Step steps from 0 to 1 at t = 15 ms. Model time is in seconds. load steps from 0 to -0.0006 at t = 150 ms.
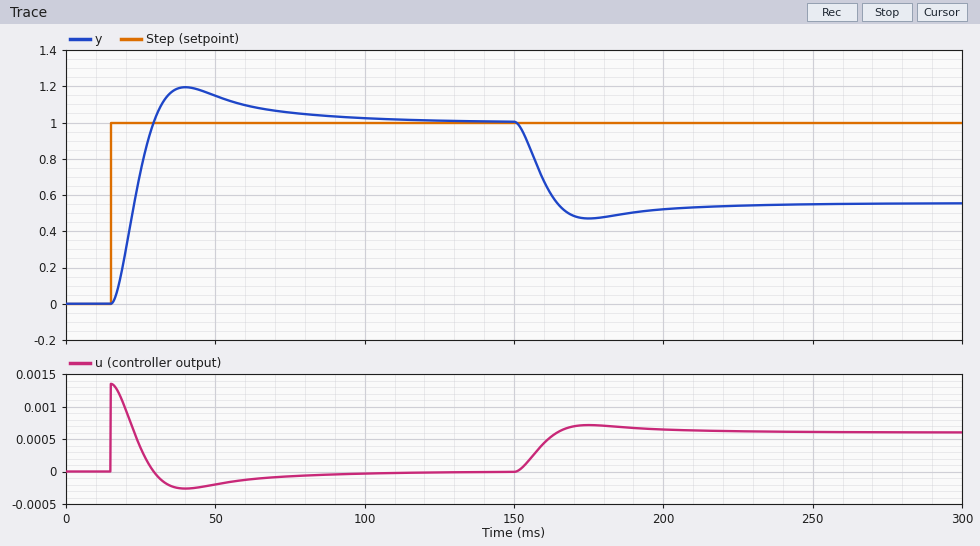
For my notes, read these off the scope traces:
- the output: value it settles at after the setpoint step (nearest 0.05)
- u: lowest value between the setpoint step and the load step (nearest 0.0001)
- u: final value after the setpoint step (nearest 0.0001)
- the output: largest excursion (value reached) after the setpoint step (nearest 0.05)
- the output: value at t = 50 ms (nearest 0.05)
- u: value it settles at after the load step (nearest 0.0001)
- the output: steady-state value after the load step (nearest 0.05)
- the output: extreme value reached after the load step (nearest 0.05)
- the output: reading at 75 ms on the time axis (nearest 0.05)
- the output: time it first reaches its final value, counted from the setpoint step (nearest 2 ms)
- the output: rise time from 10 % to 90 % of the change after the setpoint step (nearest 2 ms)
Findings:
1.00
-0.0003
0.0000
1.20
1.15
0.0006
0.55
0.45
1.05
14 ms
10 ms
